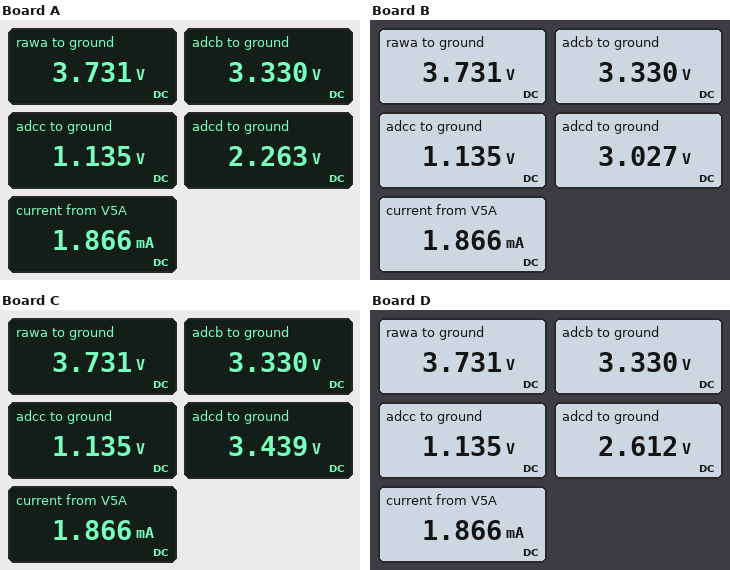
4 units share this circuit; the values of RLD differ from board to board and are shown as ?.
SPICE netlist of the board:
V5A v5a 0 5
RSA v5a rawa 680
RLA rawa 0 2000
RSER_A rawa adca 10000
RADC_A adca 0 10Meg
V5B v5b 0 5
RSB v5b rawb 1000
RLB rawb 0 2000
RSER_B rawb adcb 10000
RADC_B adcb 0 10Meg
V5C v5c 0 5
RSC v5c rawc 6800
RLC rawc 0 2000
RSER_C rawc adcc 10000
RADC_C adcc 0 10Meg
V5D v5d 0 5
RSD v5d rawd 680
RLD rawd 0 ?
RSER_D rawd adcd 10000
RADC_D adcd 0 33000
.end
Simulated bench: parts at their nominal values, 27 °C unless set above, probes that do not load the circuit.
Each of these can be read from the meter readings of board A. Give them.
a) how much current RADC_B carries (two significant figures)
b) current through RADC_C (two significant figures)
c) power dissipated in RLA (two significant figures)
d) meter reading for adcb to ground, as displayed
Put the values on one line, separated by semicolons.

330 nA; 110 nA; 7.0 mW; 3.330 V
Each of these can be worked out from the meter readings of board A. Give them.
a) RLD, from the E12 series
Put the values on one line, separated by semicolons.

1 kΩ
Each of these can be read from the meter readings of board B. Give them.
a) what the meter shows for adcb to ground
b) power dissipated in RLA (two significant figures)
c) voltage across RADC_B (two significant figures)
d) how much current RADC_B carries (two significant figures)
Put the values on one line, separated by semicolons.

3.330 V; 7.0 mW; 3.3 V; 330 nA
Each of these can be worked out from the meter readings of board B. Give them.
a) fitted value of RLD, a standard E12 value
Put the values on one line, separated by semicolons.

2.7 kΩ
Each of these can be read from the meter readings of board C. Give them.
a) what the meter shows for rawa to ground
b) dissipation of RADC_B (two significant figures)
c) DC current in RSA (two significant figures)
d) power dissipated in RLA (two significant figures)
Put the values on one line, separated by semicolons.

3.731 V; 1.1 µW; 1.9 mA; 7.0 mW
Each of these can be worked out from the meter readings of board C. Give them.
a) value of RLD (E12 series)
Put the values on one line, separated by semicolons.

6.8 kΩ
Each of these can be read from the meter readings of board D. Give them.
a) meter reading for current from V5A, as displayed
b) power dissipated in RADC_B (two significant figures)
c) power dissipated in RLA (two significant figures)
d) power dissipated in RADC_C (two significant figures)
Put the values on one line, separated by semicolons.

1.866 mA; 1.1 µW; 7.0 mW; 130 nW
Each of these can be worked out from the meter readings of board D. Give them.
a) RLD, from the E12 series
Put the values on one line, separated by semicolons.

1.5 kΩ
